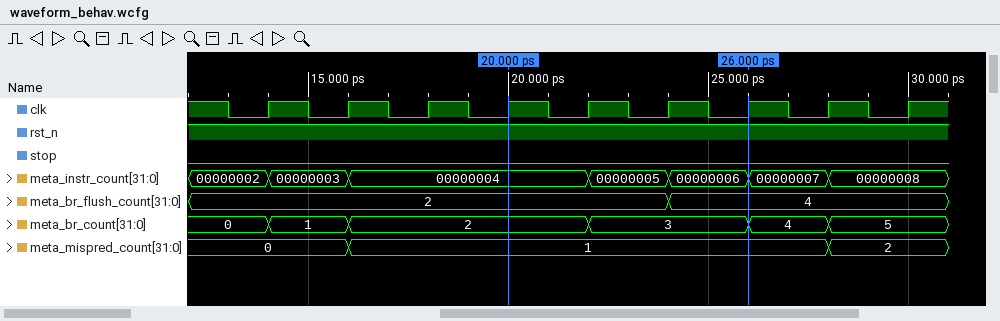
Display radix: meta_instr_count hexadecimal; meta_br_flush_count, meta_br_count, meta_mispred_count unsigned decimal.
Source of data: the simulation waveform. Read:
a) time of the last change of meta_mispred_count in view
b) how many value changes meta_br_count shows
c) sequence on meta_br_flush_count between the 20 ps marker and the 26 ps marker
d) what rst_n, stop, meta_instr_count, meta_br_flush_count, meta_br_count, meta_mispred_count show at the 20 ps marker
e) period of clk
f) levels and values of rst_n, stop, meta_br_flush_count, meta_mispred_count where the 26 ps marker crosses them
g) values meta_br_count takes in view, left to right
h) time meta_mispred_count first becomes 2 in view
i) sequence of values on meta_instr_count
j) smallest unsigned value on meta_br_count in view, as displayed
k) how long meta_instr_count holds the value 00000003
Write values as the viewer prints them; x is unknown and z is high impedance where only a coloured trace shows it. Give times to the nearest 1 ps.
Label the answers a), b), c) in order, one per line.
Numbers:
a) 28 ps
b) 5
c) 2, 4
d) rst_n=1, stop=0, meta_instr_count=00000004, meta_br_flush_count=2, meta_br_count=2, meta_mispred_count=1
e) 2 ps
f) rst_n=1, stop=0, meta_br_flush_count=4, meta_mispred_count=1
g) 0, 1, 2, 3, 4, 5
h) 28 ps
i) 00000002, 00000003, 00000004, 00000005, 00000006, 00000007, 00000008
j) 0
k) 2 ps
